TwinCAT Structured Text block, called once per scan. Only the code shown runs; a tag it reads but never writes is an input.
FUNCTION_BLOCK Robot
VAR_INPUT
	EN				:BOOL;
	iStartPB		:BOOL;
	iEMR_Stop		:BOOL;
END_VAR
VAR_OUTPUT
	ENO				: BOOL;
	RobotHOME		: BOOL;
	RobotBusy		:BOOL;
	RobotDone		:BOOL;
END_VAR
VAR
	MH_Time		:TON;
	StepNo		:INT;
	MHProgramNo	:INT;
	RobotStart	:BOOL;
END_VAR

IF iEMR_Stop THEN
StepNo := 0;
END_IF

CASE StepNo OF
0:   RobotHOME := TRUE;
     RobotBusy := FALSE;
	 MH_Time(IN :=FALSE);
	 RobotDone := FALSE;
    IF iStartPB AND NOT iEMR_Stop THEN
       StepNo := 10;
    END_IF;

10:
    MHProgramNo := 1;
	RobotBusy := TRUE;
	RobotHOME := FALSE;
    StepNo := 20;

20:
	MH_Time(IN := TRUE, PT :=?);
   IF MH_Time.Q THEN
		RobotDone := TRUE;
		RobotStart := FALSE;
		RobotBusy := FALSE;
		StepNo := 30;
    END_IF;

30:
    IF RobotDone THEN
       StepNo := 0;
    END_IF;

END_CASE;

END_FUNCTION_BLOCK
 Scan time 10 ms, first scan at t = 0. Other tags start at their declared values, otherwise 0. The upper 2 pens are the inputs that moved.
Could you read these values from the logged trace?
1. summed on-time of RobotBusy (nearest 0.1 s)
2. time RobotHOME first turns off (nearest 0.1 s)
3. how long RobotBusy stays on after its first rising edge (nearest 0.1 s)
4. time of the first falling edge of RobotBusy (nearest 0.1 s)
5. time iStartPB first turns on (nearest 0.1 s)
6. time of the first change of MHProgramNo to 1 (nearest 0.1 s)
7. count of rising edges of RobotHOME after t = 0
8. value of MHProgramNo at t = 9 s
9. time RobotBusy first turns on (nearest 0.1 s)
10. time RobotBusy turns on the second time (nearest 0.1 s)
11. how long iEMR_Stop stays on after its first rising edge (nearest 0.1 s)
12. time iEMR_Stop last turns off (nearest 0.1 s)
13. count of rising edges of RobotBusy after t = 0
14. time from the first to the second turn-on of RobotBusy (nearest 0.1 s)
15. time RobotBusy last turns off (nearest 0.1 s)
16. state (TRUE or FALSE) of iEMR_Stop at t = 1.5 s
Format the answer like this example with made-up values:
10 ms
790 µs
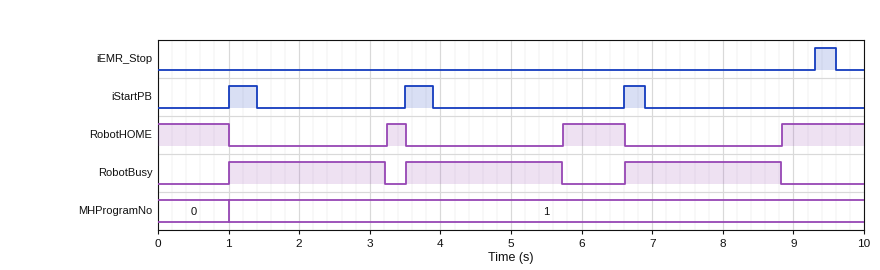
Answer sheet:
6.6 s
1.0 s
2.2 s
3.2 s
1.0 s
1.0 s
3
1
1.0 s
3.5 s
0.3 s
9.6 s
3
2.5 s
8.8 s
FALSE
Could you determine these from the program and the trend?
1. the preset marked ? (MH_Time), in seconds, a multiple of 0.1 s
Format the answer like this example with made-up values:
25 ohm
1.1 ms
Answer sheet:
2.2 s
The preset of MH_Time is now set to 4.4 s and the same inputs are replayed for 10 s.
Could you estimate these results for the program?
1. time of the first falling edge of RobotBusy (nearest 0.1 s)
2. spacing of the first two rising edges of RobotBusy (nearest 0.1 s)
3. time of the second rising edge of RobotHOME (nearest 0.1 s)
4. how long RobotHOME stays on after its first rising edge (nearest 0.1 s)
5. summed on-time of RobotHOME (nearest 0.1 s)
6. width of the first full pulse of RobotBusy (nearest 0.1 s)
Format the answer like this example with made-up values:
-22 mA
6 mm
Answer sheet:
5.4 s
5.6 s
9.3 s
1.2 s
2.9 s
4.4 s
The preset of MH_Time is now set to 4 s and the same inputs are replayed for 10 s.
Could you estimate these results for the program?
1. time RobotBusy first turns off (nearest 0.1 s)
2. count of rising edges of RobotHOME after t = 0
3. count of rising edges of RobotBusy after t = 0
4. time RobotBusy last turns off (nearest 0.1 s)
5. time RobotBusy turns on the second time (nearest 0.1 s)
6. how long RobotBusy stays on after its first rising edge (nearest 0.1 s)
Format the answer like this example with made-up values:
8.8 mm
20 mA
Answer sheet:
5.0 s
2
2
9.3 s
6.6 s
4.0 s
